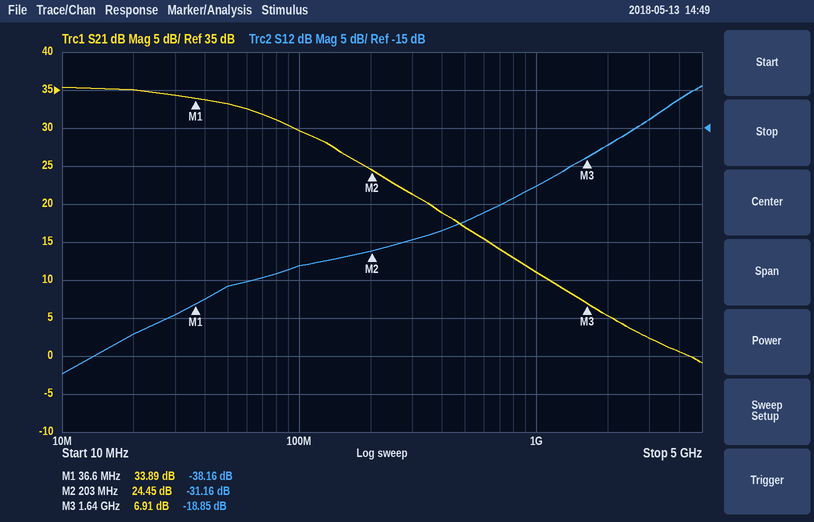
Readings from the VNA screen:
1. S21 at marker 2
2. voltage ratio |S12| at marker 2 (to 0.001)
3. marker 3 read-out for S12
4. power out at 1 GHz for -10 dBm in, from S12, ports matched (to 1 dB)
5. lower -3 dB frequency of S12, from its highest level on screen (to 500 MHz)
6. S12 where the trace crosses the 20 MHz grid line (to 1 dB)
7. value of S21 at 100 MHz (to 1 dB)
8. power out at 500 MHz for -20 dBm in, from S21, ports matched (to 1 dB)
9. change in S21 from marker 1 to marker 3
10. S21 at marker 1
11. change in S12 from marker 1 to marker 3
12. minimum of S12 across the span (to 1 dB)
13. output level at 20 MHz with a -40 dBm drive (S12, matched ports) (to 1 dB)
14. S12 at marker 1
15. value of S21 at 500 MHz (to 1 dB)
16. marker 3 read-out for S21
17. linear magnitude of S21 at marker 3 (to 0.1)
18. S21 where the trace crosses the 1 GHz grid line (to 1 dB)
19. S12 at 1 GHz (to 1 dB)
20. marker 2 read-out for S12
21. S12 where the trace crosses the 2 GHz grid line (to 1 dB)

24.45 dB
0.028
-18.85 dB
-33 dBm
3.5 GHz
-42 dB
30 dB
-3 dBm
-26.98 dB
33.89 dB
19.31 dB
-47 dB
-82 dBm
-38.16 dB
17 dB
6.91 dB
2.2
11 dB
-23 dB
-31.16 dB
-17 dB
